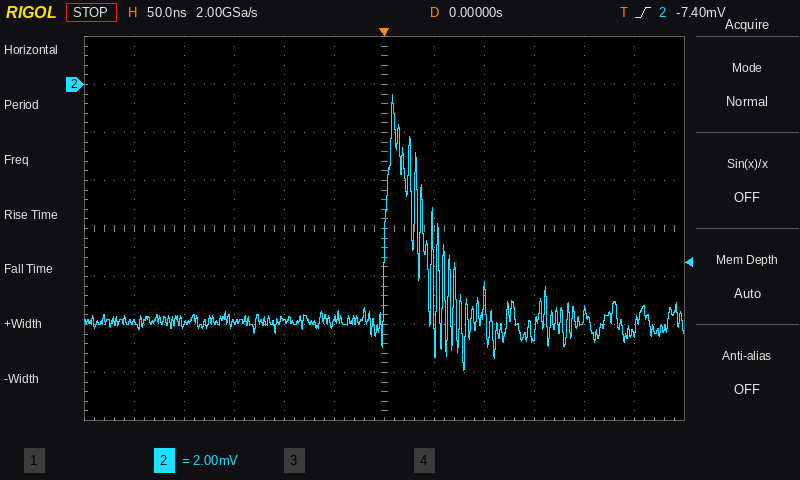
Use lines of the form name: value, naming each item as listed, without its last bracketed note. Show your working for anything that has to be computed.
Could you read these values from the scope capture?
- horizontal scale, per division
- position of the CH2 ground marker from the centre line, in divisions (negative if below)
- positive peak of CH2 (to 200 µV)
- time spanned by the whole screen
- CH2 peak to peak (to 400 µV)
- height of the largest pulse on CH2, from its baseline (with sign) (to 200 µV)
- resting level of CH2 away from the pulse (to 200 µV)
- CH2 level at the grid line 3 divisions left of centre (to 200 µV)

horizontal scale, per division: 50 ns
position of the CH2 ground marker from the centre line, in divisions: +3.0 div
positive peak of CH2: -400 µV
time spanned by the whole screen: 600 ns
CH2 peak to peak: 11.6 mV
height of the largest pulse on CH2, from its baseline (with sign): -400 µV − (-9.8 mV) = +9.4 mV
resting level of CH2 away from the pulse: -9.8 mV
CH2 level at the grid line 3 divisions left of centre: -10.0 mV
